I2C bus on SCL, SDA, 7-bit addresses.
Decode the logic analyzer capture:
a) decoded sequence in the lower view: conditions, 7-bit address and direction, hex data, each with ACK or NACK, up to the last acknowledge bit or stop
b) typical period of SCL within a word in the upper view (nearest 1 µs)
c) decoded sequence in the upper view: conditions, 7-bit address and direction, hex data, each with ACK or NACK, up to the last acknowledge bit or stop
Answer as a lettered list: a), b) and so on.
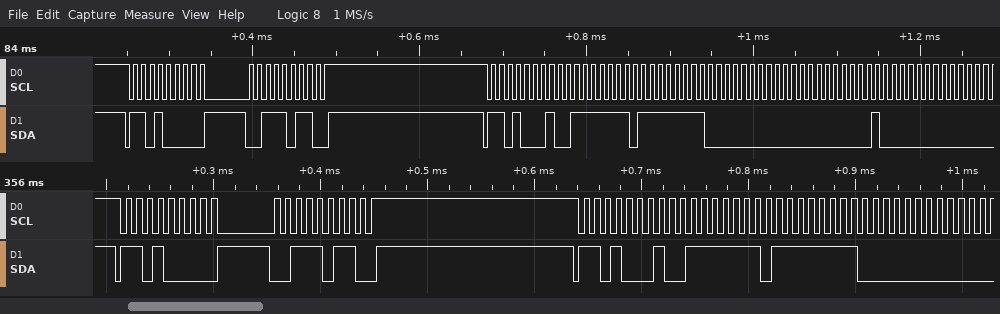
a) start, address 68 write ACK, 3B ACK, stop, start, address 68 read ACK, 7F ACK, FF ACK, 00 ACK
b) 10 µs
c) start, address 68 write ACK, 3B ACK, stop, start, address 68 read ACK, 7F ACK, FF ACK, 00 ACK, 00 ACK, 40 ACK
